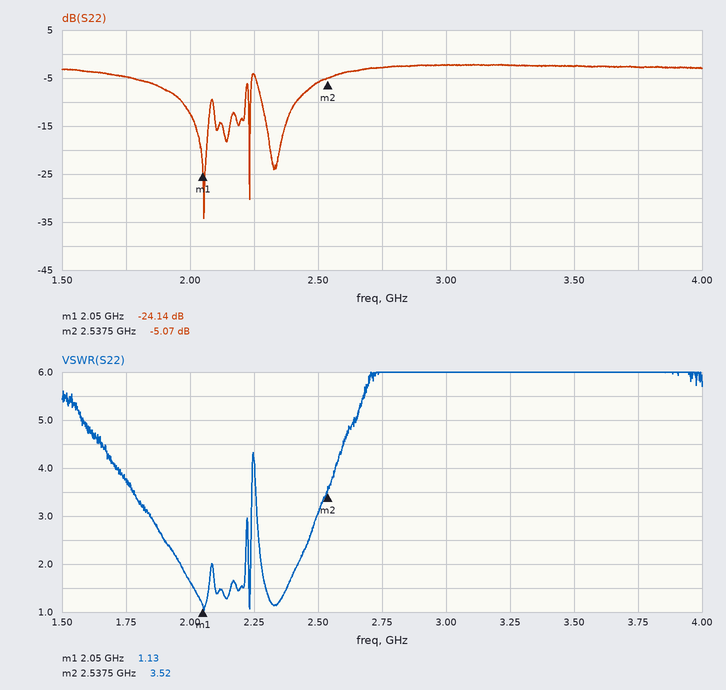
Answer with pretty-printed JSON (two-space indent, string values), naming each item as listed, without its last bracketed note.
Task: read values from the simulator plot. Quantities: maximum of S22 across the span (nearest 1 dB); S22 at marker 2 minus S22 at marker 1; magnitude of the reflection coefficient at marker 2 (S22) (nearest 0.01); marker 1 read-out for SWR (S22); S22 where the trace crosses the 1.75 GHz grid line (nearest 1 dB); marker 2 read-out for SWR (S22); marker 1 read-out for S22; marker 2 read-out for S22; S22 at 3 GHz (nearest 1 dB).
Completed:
{
  "maximum of S22 across the span": "-2 dB",
  "S22 at marker 2 minus S22 at marker 1": "19.07 dB",
  "magnitude of the reflection coefficient at marker 2 (S22)": "0.56",
  "marker 1 read-out for SWR": "1.13",
  "S22 where the trace crosses the 1.75 GHz grid line": "-5 dB",
  "marker 2 read-out for SWR": "3.52",
  "marker 1 read-out for S22": "-24.14 dB",
  "marker 2 read-out for S22": "-5.07 dB",
  "S22 at 3 GHz": "-2 dB"
}
